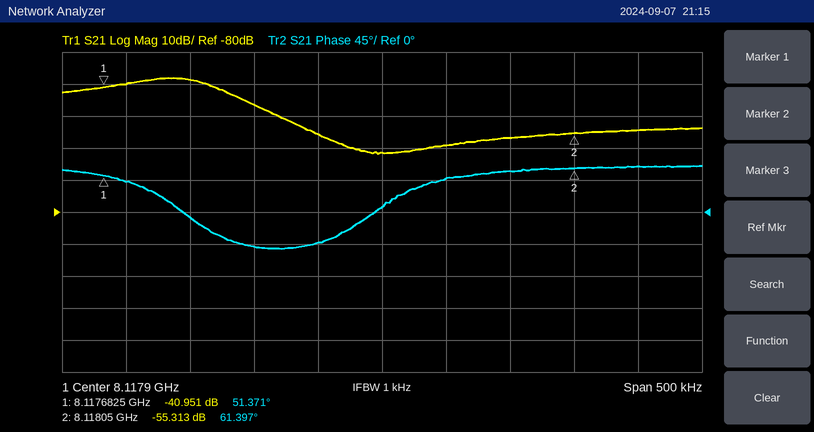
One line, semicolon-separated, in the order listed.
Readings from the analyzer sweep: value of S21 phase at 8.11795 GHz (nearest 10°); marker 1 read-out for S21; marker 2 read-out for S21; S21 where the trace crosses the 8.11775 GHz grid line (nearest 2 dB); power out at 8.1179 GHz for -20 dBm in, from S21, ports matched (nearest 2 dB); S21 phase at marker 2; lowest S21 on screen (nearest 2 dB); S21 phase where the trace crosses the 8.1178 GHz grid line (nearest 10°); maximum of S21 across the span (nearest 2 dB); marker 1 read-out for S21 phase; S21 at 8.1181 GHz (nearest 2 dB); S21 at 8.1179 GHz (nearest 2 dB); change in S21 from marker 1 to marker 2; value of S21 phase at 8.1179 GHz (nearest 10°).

50°; -40.951 dB; -55.313 dB; -38 dB; -82 dBm; 61.397°; -62 dB; -50°; -38 dB; 51.371°; -54 dB; -62 dB; -14.362 dB; 10°
